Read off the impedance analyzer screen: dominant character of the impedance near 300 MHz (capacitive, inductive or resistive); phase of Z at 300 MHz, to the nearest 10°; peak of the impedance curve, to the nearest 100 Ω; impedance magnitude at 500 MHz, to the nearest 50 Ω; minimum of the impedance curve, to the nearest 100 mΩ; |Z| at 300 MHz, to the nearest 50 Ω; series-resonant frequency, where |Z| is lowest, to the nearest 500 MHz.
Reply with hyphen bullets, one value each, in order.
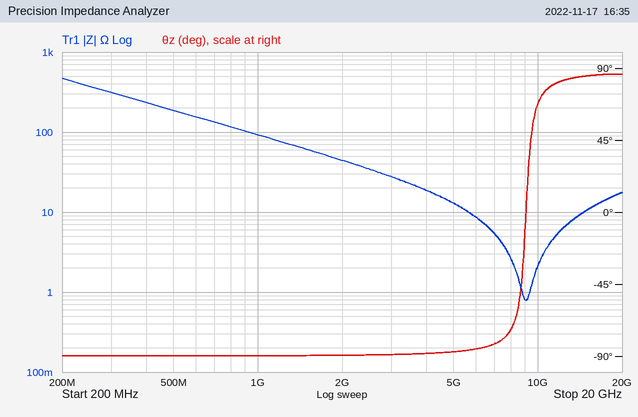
- capacitive
- -90°
- 500 Ω
- 200 Ω
- 800 mΩ
- 300 Ω
- 9.0 GHz
